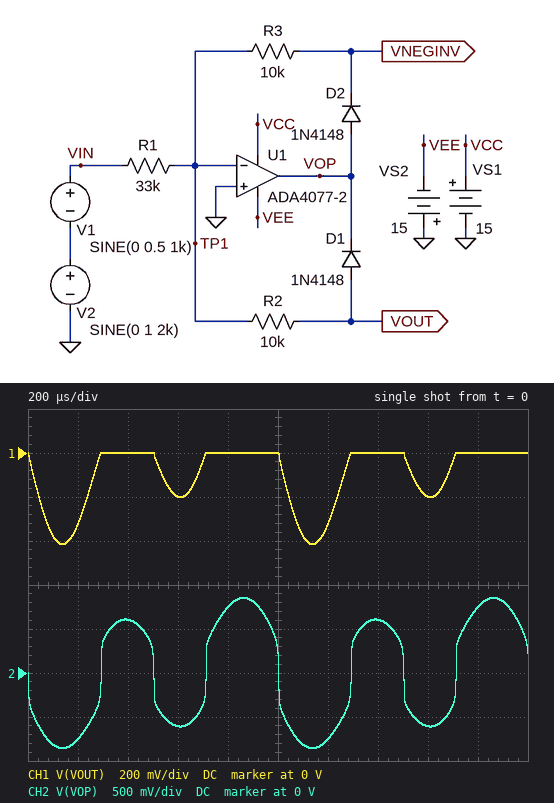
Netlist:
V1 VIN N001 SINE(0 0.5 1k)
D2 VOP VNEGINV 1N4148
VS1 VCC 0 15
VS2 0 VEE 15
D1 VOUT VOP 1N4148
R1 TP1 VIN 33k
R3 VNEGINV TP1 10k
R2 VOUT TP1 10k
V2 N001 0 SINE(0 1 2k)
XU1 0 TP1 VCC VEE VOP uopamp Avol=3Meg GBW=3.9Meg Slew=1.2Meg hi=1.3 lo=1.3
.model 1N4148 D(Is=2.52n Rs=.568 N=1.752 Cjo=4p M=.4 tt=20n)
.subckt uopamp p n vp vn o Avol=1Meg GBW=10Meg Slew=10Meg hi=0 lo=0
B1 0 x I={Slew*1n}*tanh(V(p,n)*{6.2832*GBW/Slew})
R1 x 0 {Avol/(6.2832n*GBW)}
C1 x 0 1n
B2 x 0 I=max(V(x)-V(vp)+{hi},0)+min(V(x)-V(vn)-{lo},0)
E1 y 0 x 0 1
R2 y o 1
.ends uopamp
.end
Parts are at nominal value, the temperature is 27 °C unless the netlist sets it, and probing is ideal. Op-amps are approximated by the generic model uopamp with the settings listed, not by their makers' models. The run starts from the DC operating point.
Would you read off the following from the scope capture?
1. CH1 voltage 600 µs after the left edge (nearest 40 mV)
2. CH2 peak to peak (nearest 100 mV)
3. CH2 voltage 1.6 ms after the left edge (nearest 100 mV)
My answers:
-200 mV
1.7 V
-600 mV
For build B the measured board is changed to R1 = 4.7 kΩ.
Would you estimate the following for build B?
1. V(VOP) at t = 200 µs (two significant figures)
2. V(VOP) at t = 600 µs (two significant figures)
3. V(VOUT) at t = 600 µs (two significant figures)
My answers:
-2.8 V
-1.9 V
-1.4 V
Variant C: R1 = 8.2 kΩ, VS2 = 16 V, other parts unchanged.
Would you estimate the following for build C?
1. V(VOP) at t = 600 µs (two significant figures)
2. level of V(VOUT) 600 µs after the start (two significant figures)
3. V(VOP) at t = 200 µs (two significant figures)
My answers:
-1.3 V
-800 mV
-1.8 V
